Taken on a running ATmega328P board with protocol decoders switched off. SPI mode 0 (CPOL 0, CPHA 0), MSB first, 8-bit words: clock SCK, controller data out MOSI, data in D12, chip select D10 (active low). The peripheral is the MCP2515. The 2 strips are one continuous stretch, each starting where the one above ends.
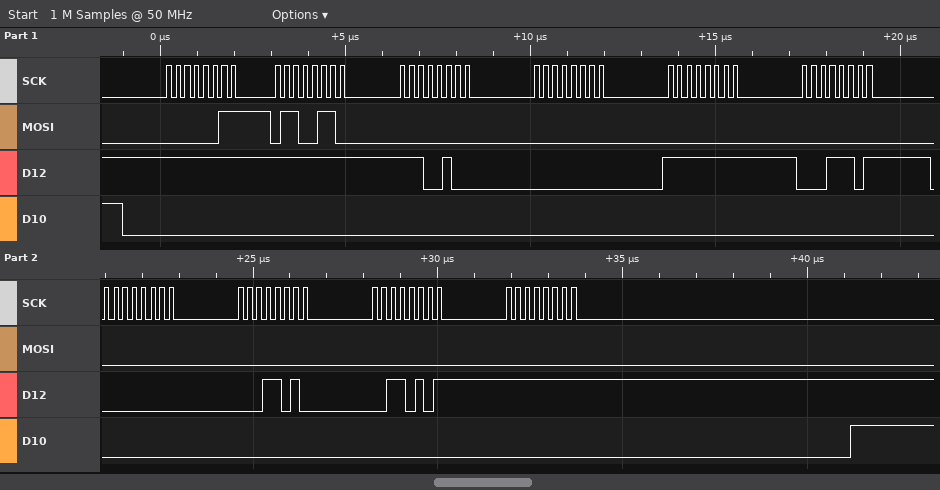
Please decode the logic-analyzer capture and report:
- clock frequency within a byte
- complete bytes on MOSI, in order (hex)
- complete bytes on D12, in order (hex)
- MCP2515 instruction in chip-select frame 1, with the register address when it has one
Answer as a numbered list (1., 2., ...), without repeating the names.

1. 4 MHz
2. 03 66 00 00 00 00 00 00 00 00
3. FF FF E4 00 FF 1D 00 1A 35 FF
4. READ 0x66
